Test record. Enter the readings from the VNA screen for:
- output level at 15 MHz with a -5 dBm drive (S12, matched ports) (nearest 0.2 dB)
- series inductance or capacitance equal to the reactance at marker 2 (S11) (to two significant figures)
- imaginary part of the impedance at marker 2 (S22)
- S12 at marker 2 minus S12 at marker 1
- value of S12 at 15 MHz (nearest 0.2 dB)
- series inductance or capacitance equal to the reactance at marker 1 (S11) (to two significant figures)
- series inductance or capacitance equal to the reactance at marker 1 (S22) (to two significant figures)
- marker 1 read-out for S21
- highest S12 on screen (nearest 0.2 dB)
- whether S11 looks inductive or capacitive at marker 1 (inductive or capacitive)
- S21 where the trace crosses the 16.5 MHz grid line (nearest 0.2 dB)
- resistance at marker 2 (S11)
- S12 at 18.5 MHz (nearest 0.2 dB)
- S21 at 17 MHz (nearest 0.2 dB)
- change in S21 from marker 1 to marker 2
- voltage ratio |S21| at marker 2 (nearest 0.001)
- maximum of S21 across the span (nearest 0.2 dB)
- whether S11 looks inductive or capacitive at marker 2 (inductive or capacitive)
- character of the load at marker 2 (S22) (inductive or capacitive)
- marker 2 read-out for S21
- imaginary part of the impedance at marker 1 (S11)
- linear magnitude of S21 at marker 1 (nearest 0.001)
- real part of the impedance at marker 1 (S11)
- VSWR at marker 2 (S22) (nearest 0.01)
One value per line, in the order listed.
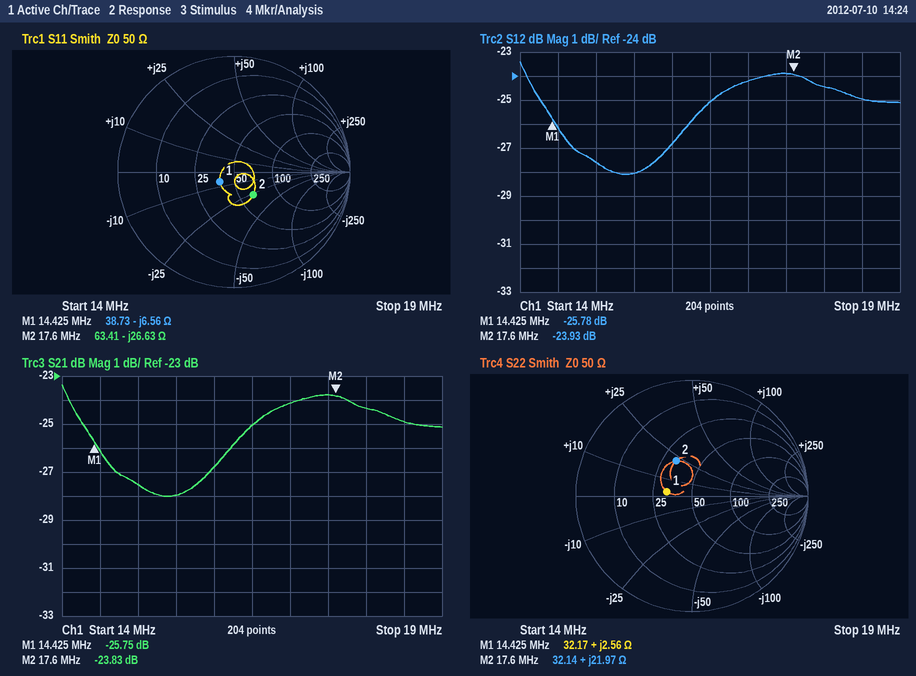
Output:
-32.6 dBm
340 pF
+21.97 Ω
1.85 dB
-27.6 dB
1.7 nF
28 nH
-25.75 dB
-23.4 dB
capacitive
-25.0 dB
63.41 Ω
-25.0 dB
-24.2 dB
1.92 dB
0.064
-23.4 dB
capacitive
inductive
-23.83 dB
-6.56 Ω
0.052
38.73 Ω
2.00
